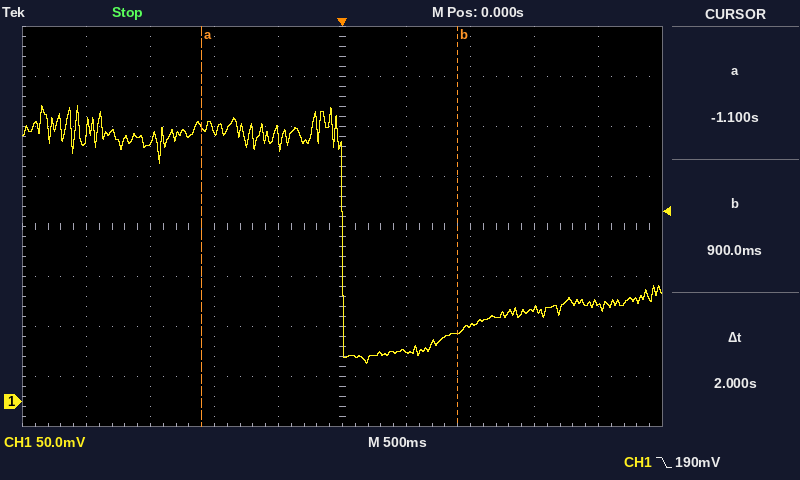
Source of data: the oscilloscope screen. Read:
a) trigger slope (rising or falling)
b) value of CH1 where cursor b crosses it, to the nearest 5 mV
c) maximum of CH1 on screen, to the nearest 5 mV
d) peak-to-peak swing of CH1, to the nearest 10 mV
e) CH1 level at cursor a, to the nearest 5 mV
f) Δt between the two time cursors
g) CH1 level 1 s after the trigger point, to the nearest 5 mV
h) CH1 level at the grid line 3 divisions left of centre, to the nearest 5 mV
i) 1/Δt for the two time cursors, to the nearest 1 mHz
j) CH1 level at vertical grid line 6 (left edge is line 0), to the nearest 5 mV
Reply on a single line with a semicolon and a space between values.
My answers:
falling; 70 mV; 295 mV; 260 mV; 275 mV; 2 s; 75 mV; 260 mV; 500 mHz; 50 mV
